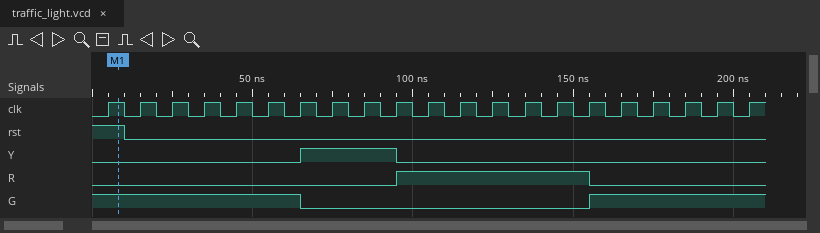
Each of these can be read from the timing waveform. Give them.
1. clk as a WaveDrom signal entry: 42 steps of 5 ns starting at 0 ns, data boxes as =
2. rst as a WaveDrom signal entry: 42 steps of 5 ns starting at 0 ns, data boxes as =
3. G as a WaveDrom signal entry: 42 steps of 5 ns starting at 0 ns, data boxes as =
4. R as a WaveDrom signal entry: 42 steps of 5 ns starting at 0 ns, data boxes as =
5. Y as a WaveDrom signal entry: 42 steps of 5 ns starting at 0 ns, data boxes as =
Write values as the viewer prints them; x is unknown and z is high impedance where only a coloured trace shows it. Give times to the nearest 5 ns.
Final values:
{name: 'clk', wave: '010101010101010101010101010101010101010101'}
{name: 'rst', wave: '1.0.......................................'}
{name: 'G', wave: '1............0.................1..........'}
{name: 'R', wave: '0..................1...........0..........'}
{name: 'Y', wave: '0............1.....0......................'}
